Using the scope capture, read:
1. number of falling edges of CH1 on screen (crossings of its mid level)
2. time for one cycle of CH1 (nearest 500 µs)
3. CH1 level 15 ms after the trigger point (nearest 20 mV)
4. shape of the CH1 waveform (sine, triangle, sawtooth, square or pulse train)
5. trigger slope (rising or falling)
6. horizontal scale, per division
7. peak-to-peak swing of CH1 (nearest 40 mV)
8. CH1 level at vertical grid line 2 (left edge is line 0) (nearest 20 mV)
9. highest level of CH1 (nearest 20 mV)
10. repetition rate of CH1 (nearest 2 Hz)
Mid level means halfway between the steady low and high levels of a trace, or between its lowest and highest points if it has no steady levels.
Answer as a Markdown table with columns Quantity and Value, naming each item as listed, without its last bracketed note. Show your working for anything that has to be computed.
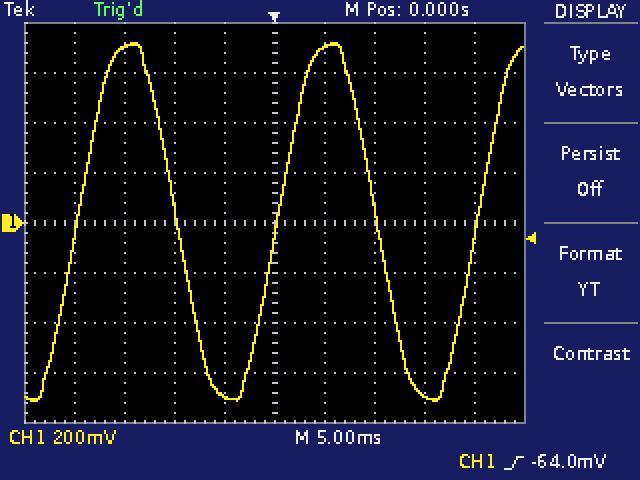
| Quantity | Value |
|---|---|
| number of falling edges of CH1 on screen | 2 |
| time for one cycle of CH1 | 20.0 ms |
| CH1 level 15 ms after the trigger point | -700 mV |
| shape of the CH1 waveform | sine |
| trigger slope | rising |
| horizontal scale, per division | 5 ms |
| peak-to-peak swing of CH1 | 1.44 V |
| CH1 level at vertical grid line 2 (left edge is line 0) | 700 mV |
| highest level of CH1 | 720 mV |
| repetition rate of CH1 | 1 / 20.0 ms ≈ 50 Hz |
